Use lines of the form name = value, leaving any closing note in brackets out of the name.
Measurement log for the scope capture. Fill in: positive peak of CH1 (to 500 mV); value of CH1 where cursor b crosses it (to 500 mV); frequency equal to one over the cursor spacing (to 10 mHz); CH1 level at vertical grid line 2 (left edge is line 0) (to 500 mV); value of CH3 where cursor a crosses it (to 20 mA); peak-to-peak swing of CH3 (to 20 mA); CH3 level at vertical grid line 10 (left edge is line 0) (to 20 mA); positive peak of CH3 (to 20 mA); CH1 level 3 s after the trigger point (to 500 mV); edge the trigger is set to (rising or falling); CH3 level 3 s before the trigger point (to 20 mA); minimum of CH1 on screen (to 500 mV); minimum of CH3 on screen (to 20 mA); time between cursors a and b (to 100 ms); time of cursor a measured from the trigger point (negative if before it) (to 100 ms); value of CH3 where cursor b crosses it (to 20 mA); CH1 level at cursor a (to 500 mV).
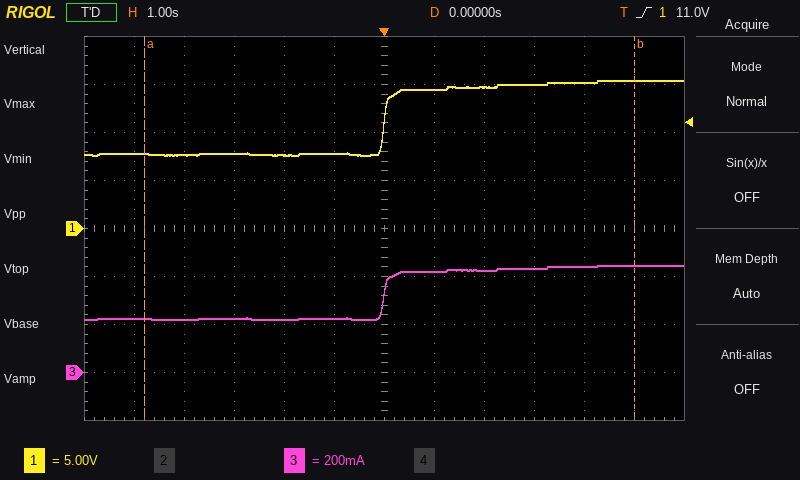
positive peak of CH1 = 15.5 V
value of CH1 where cursor b crosses it = 15.5 V
frequency equal to one over the cursor spacing = 100 mHz
CH1 level at vertical grid line 2 (left edge is line 0) = 7.5 V
value of CH3 where cursor a crosses it = 220 mA
peak-to-peak swing of CH3 = 220 mA
CH3 level at vertical grid line 10 (left edge is line 0) = 440 mA
positive peak of CH3 = 440 mA
CH1 level 3 s after the trigger point = 15.0 V
edge the trigger is set to = rising
CH3 level 3 s before the trigger point = 220 mA
minimum of CH1 on screen = 7.5 V
minimum of CH3 on screen = 220 mA
time between cursors a and b = 9.8 s
time of cursor a measured from the trigger point (negative if before it) = -4.8 s
value of CH3 where cursor b crosses it = 440 mA
CH1 level at cursor a = 8.0 V
